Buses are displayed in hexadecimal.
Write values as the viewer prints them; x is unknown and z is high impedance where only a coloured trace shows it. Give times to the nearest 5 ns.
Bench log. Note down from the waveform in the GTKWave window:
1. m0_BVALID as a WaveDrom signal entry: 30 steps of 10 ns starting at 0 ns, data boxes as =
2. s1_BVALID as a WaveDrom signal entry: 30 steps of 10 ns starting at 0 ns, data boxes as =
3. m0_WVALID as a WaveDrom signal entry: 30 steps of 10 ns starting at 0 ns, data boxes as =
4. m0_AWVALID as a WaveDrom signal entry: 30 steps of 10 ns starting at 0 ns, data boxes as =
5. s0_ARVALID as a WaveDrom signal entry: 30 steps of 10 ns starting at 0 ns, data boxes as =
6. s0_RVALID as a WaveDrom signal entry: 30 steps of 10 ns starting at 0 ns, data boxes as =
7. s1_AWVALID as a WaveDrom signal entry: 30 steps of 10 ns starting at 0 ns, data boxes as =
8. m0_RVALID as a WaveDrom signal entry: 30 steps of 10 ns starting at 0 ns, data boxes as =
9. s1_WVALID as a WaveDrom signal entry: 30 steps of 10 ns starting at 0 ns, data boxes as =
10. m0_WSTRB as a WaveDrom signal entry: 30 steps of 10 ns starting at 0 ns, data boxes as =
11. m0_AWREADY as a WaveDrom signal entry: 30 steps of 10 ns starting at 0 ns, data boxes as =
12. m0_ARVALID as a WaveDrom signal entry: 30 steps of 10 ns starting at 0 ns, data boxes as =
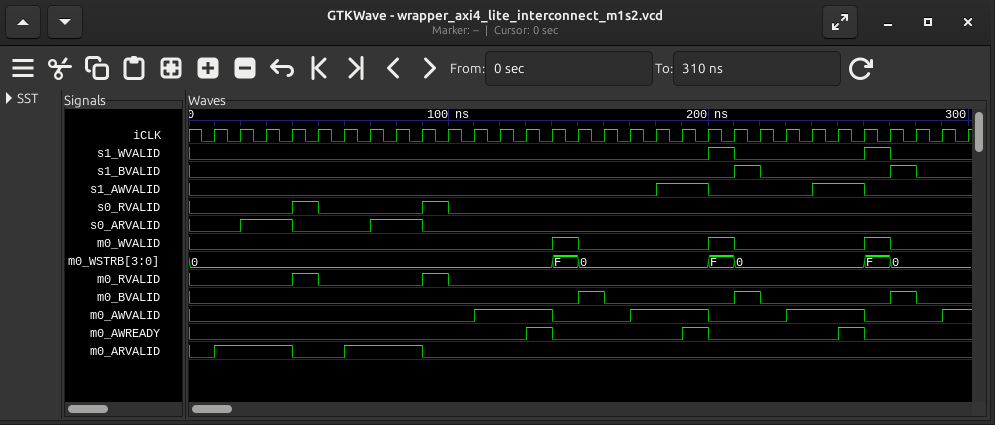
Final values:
{name: 'm0_BVALID', wave: '0..............10....10....10.'}
{name: 's1_BVALID', wave: '0....................10....10.'}
{name: 'm0_WVALID', wave: '0.............10....10....10..'}
{name: 'm0_AWVALID', wave: '0..........1..0..1..0..1..0..1'}
{name: 's0_ARVALID', wave: '0.1.0..1.0....................'}
{name: 's0_RVALID', wave: '0...10...10...................'}
{name: 's1_AWVALID', wave: '0.................1.0...1.0...'}
{name: 'm0_RVALID', wave: '0...10...10...................'}
{name: 's1_WVALID', wave: '0...................10....10..'}
{name: 'm0_WSTRB', wave: '=.............==....==....==..', data: '0 F 0 F 0 F 0'}
{name: 'm0_AWREADY', wave: '0............10....10....10...'}
{name: 'm0_ARVALID', wave: '01..0.1..0....................'}
